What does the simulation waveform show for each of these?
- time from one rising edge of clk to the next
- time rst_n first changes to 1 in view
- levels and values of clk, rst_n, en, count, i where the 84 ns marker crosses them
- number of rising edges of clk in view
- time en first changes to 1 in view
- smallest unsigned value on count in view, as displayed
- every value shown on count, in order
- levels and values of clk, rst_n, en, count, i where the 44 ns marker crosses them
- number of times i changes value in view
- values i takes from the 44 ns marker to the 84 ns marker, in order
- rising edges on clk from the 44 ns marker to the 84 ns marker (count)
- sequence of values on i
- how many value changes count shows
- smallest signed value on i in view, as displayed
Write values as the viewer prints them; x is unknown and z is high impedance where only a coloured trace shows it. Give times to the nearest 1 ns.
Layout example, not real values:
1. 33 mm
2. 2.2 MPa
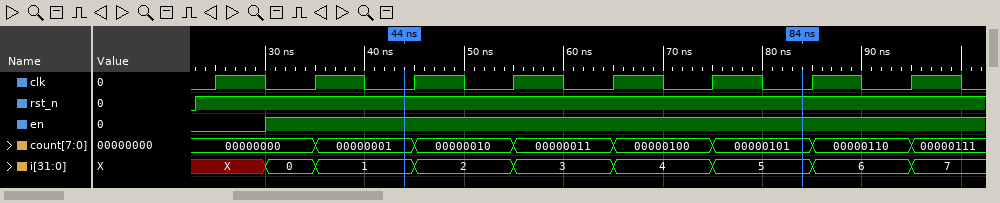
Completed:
1. 10 ns
2. 23 ns
3. clk=0, rst_n=1, en=1, count=00000101, i=5
4. 8
5. 30 ns
6. 00000000
7. 00000000, 00000001, 00000010, 00000011, 00000100, 00000101, 00000110, 00000111
8. clk=0, rst_n=1, en=1, count=00000001, i=1
9. 8
10. 1, 2, 3, 4, 5
11. 4
12. X, 0, 1, 2, 3, 4, 5, 6, 7
13. 7
14. 0
